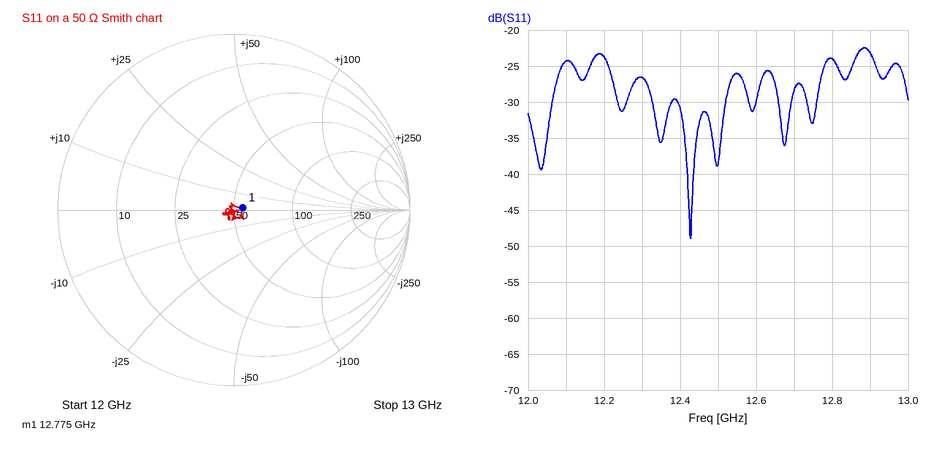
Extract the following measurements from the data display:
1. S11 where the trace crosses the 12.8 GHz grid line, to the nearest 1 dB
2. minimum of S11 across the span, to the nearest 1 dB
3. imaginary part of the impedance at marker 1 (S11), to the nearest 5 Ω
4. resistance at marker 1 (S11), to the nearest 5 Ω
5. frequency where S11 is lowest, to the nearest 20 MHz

-24 dB
-49 dB
0 Ω
55 Ω
12.42 GHz
